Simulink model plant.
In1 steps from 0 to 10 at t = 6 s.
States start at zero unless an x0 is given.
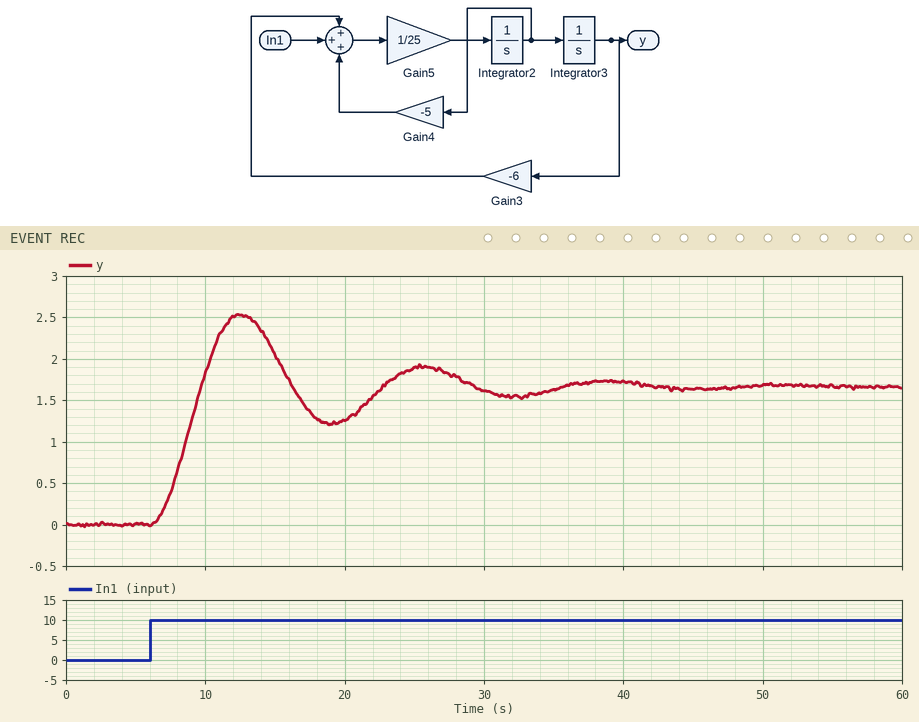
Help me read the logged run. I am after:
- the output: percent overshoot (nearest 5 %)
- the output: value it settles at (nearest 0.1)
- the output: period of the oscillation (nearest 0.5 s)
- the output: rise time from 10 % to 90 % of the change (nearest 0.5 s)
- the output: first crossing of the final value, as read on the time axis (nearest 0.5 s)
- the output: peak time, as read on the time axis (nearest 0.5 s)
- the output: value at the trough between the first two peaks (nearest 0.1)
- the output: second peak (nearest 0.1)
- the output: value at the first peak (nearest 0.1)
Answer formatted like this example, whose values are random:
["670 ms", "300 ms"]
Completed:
["50 %", "1.7", "13.0 s", "2.5 s", "9.5 s", "12.5 s", "1.2", "1.9", "2.5"]
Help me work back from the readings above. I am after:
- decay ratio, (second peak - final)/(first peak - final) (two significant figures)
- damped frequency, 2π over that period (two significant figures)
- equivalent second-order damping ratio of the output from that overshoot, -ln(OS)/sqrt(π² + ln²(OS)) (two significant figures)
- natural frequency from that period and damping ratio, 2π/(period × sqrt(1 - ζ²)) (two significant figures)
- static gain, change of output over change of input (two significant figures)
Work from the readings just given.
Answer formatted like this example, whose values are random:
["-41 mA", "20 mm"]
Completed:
["0.25", "0.48 rad/s", "0.22", "0.50 rad/s", "0.17"]
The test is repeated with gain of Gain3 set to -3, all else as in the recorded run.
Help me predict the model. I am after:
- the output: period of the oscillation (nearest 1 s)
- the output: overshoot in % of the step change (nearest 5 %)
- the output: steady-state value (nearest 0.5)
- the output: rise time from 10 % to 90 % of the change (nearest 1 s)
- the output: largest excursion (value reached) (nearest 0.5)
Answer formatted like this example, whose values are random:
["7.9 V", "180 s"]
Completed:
["19 s", "40 %", "3.5", "4 s", "4.5"]
